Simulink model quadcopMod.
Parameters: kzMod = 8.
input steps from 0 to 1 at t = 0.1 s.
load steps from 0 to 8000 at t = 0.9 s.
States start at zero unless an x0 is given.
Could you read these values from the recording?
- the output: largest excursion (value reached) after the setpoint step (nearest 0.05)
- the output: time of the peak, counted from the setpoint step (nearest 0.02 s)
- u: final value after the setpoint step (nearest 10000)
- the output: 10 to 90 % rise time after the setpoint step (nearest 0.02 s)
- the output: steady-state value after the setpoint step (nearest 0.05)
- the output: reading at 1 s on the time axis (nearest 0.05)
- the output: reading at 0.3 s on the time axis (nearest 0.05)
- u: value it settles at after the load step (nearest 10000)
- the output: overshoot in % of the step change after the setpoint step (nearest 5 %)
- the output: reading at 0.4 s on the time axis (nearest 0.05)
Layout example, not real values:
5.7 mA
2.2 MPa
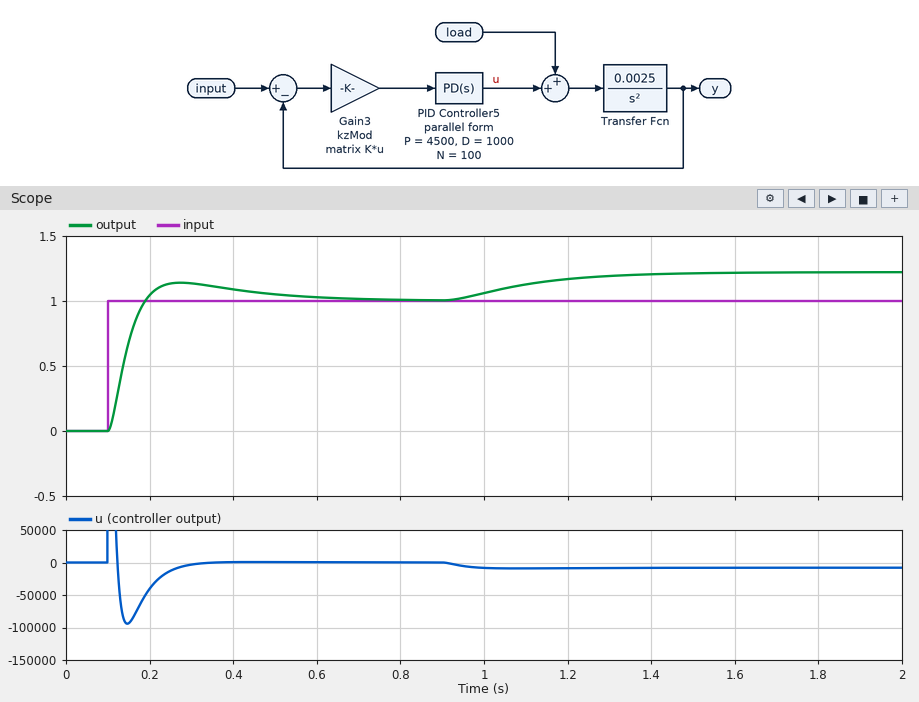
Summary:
1.15
0.18 s
0
0.06 s
1.00
1.05
1.15
-10000
15 %
1.10
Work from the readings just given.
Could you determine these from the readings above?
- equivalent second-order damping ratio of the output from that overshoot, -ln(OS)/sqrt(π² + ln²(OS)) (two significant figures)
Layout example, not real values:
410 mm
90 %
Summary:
0.52
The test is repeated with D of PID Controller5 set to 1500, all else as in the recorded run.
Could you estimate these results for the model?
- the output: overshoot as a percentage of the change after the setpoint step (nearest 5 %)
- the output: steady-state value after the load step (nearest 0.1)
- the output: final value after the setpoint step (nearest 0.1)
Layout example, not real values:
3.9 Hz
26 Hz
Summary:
10 %
1.2
1.0
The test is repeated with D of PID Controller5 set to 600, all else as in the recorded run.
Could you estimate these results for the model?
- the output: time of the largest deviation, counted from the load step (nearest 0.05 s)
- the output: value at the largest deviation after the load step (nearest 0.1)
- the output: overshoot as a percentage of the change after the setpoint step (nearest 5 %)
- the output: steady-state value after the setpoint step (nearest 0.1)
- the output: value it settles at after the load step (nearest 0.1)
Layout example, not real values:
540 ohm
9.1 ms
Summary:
0.40 s
1.2
25 %
1.0
1.2
